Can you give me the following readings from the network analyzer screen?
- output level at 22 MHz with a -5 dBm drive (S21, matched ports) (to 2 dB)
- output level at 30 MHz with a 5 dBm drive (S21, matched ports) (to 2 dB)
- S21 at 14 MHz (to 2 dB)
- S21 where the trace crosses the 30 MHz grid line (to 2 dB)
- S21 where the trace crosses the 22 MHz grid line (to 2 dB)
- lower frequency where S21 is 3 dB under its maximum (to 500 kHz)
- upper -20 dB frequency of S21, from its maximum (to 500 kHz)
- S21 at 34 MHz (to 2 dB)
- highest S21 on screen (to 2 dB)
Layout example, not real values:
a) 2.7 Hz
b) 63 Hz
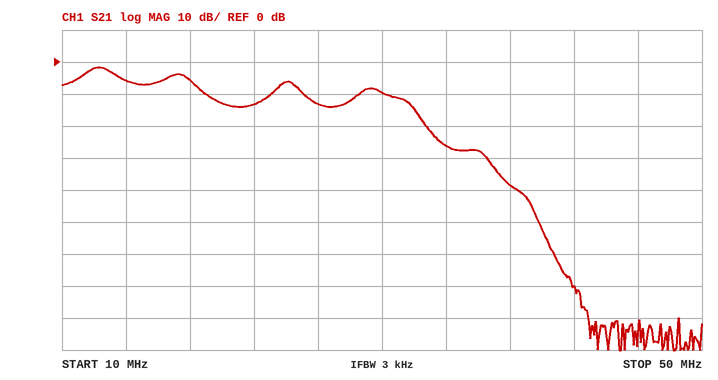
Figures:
a) -18 dBm
b) -4 dBm
c) -6 dB
d) -10 dB
e) -14 dB
f) 11.0 MHz
g) 33.0 MHz
h) -26 dB
i) -2 dB
